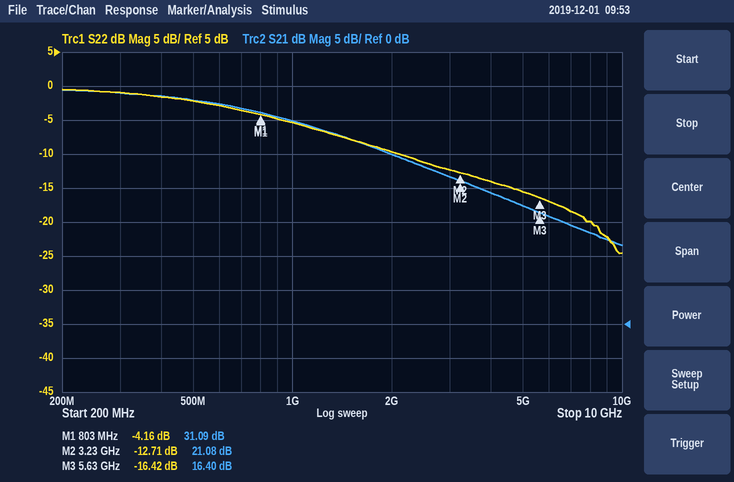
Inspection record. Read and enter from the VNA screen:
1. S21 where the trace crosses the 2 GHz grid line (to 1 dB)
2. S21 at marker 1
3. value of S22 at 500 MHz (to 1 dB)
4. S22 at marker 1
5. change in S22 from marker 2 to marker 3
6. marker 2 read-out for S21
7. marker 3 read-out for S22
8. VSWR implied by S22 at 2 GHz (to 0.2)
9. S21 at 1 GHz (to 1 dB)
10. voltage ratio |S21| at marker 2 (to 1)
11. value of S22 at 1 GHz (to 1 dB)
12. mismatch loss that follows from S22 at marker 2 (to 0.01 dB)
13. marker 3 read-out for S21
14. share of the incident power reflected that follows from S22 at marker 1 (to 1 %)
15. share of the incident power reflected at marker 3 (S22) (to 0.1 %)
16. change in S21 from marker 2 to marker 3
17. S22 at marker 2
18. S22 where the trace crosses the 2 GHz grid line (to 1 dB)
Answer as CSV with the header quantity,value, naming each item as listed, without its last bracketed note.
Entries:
quantity,value
S21 where the trace crosses the 2 GHz grid line,25 dB
S21 at marker 1,31.09 dB
value of S22 at 500 MHz,-2 dB
S22 at marker 1,-4.16 dB
change in S22 from marker 2 to marker 3,-3.71 dB
marker 2 read-out for S21,21.08 dB
marker 3 read-out for S22,-16.42 dB
VSWR implied by S22 at 2 GHz,2.0
S21 at 1 GHz,30 dB
voltage ratio |S21| at marker 2,11
value of S22 at 1 GHz,-5 dB
mismatch loss that follows from S22 at marker 2,0.24 dB
marker 3 read-out for S21,16.40 dB
share of the incident power reflected that follows from S22 at marker 1,38 %
share of the incident power reflected at marker 3 (S22),2.3 %
change in S21 from marker 2 to marker 3,-4.68 dB
S22 at marker 2,-12.71 dB
S22 where the trace crosses the 2 GHz grid line,-10 dB
